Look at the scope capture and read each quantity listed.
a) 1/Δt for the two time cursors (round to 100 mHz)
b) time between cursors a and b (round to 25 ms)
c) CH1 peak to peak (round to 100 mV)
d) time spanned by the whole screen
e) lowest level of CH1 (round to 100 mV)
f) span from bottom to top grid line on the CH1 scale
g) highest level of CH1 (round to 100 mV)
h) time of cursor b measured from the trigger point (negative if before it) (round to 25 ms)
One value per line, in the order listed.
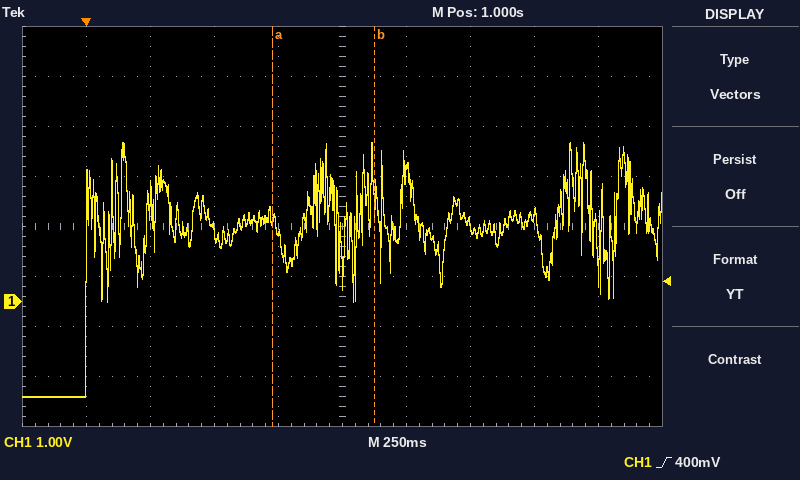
2.5 Hz
400 ms
5.1 V
2.5 s
-1.9 V
8 V
3.2 V
+1.125 s
